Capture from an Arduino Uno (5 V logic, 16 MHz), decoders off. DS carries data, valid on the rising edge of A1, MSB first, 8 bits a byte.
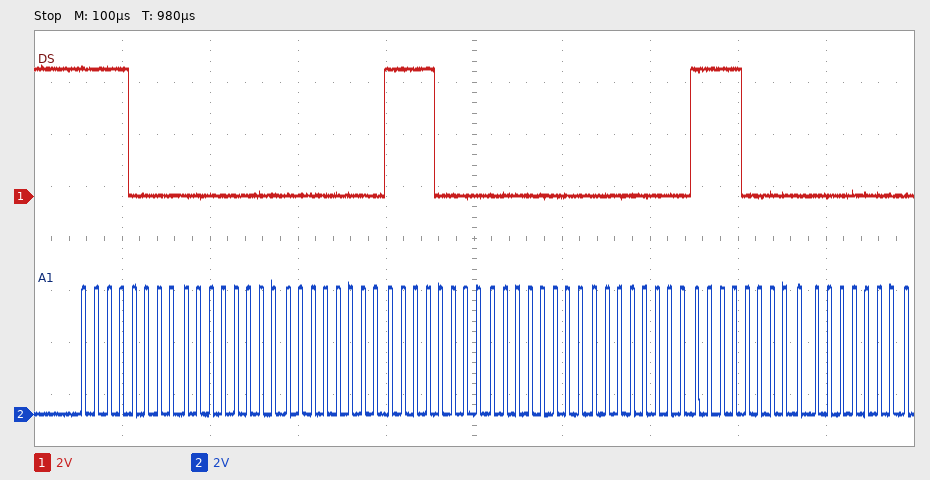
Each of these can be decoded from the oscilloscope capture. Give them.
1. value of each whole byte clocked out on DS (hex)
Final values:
0xF0 0x00 0x00 0xF0 0x00 0x00 0xF0 0x00
